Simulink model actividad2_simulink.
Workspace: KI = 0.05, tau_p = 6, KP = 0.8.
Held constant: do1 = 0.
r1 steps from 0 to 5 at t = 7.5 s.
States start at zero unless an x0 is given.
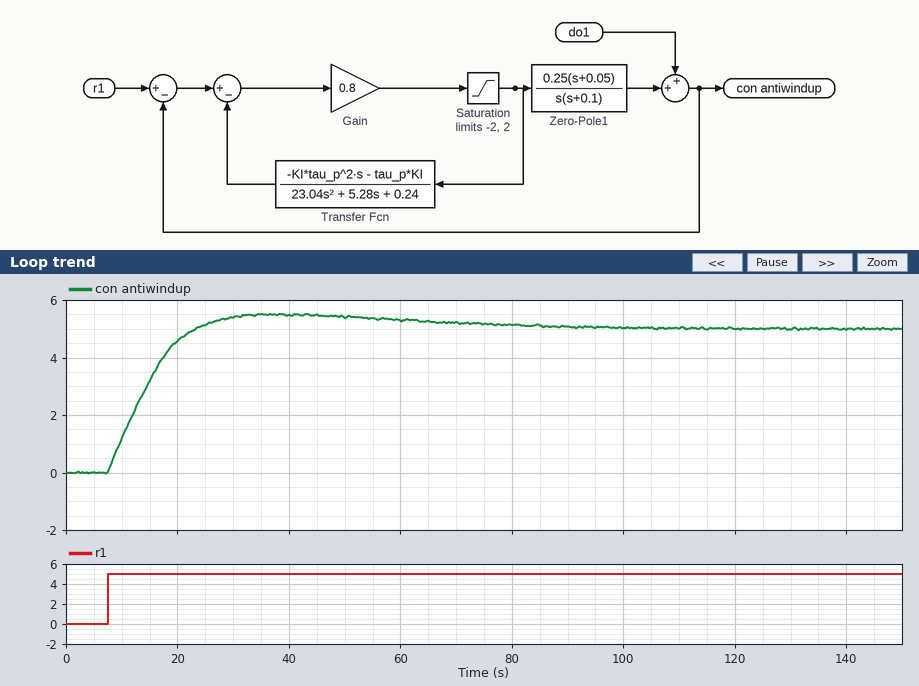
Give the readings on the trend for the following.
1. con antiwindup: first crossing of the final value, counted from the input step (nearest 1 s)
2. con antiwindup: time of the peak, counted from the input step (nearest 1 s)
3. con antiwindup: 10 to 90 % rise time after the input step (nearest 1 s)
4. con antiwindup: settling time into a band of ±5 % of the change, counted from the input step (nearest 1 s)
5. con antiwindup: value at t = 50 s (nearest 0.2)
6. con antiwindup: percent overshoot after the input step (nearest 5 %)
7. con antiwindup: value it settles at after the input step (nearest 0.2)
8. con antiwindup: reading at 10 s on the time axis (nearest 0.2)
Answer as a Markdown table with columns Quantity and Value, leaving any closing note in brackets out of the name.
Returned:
| Quantity | Value |
|---|---|
| con antiwindup: first crossing of the final value, counted from the input step | 16 s |
| con antiwindup: time of the peak, counted from the input step | 31 s |
| con antiwindup: 10 to 90 % rise time after the input step | 11 s |
| con antiwindup: settling time into a band of ±5 % of the change, counted from the input step | 58 s |
| con antiwindup: value at t = 50 s | 5.4 |
| con antiwindup: percent overshoot after the input step | 10 % |
| con antiwindup: value it settles at after the input step | 5.0 |
| con antiwindup: reading at 10 s on the time axis | 1.2 |
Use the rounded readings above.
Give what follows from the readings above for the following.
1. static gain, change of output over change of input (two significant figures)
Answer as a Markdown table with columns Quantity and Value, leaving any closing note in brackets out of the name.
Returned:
| Quantity | Value |
|---|---|
| static gain, change of output over change of input | 1.0 |
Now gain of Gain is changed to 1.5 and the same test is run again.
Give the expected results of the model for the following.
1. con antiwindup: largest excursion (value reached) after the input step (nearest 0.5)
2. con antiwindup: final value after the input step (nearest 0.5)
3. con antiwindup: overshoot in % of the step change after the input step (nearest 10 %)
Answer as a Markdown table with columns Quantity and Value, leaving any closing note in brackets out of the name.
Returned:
| Quantity | Value |
|---|---|
| con antiwindup: largest excursion (value reached) after the input step | 6.0 |
| con antiwindup: final value after the input step | 5.0 |
| con antiwindup: overshoot in % of the step change after the input step | 20 % |
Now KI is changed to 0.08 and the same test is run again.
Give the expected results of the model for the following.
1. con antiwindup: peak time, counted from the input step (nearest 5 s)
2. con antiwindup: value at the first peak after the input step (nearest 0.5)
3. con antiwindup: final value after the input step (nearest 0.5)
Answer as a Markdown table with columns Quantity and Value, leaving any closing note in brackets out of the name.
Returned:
| Quantity | Value |
|---|---|
| con antiwindup: peak time, counted from the input step | 25 s |
| con antiwindup: value at the first peak after the input step | 5.5 |
| con antiwindup: final value after the input step | 5.0 |
